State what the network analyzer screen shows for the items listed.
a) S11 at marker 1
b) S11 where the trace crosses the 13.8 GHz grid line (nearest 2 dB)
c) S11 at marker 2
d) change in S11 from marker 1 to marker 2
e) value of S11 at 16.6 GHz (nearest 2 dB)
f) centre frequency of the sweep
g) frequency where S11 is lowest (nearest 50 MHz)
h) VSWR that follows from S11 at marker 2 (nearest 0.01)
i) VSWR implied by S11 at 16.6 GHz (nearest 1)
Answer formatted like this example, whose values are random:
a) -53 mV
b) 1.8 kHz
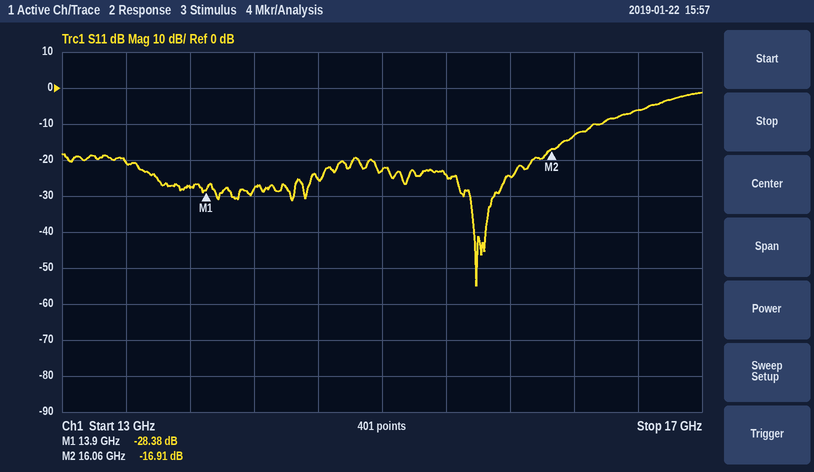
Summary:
a) -28.38 dB
b) -28 dB
c) -16.91 dB
d) 11.47 dB
e) -6 dB
f) 15 GHz
g) 15.60 GHz
h) 1.33
i) 3
